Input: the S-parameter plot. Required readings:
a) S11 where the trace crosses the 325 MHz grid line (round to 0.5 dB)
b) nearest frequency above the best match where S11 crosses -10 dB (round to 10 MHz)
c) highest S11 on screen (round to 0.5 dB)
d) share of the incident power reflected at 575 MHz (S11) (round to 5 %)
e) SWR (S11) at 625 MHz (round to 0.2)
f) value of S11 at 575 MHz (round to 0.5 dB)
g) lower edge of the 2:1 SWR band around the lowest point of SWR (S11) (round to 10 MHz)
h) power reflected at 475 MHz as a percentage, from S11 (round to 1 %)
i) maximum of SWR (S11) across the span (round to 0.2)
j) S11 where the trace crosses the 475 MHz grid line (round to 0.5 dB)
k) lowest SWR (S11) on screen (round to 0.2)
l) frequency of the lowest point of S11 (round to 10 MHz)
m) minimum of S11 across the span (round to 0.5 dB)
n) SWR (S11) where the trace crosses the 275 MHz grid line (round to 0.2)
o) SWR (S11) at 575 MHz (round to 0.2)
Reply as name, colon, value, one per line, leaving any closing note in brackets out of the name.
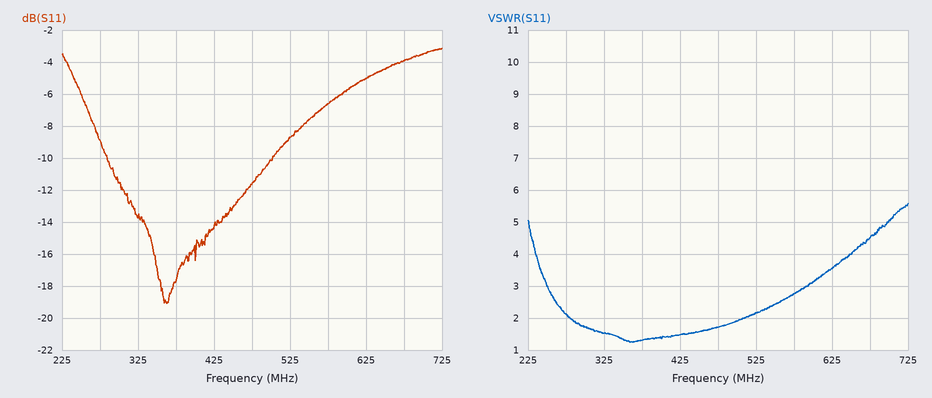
S11 where the trace crosses the 325 MHz grid line: -13.5 dB
nearest frequency above the best match where S11 crosses -10 dB: 500 MHz
highest S11 on screen: -3.0 dB
share of the incident power reflected at 575 MHz (S11): 20 %
SWR (S11) at 625 MHz: 3.6
value of S11 at 575 MHz: -6.5 dB
lower edge of the 2:1 SWR band around the lowest point of SWR (S11): 280 MHz
power reflected at 475 MHz as a percentage, from S11: 7 %
maximum of SWR (S11) across the span: 5.6
S11 where the trace crosses the 475 MHz grid line: -11.5 dB
lowest SWR (S11) on screen: 1.2
frequency of the lowest point of S11: 360 MHz
minimum of S11 across the span: -19.0 dB
SWR (S11) where the trace crosses the 275 MHz grid line: 2.2
SWR (S11) at 575 MHz: 2.8
